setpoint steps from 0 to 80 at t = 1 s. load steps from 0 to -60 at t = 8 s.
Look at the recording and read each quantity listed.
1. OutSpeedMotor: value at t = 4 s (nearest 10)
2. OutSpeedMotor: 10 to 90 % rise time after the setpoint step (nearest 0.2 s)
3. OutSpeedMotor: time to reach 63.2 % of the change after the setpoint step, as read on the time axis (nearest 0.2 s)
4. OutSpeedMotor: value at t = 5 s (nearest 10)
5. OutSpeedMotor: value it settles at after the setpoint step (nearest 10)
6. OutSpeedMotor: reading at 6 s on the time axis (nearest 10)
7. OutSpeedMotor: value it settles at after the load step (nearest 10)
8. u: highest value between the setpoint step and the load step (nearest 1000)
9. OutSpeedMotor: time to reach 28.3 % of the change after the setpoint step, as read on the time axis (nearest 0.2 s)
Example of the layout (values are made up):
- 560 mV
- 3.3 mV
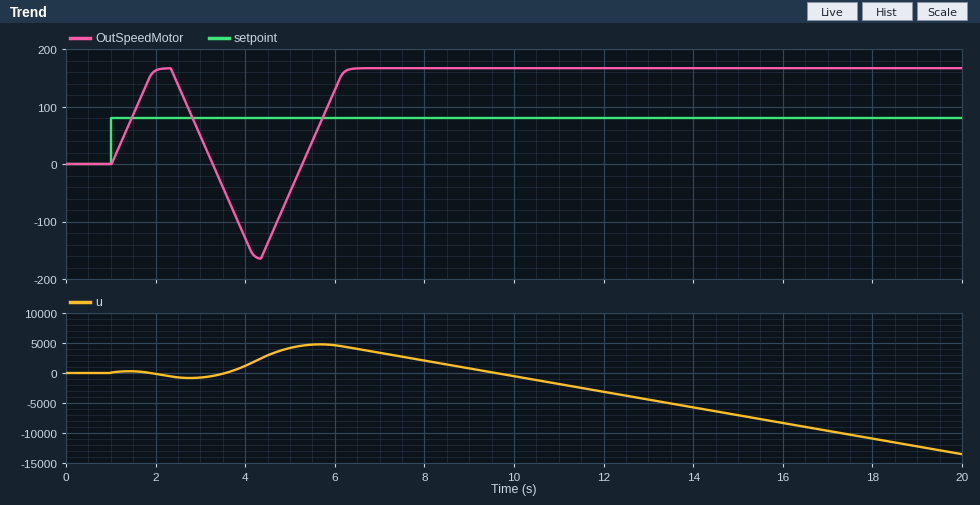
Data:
- -130
- 0.8 s
- 1.6 s
- -50
- 170
- 130
- 170
- 5000
- 1.2 s
